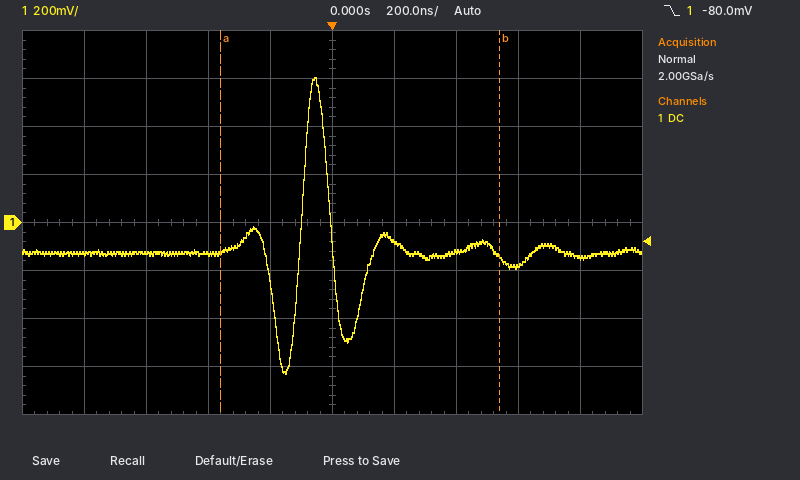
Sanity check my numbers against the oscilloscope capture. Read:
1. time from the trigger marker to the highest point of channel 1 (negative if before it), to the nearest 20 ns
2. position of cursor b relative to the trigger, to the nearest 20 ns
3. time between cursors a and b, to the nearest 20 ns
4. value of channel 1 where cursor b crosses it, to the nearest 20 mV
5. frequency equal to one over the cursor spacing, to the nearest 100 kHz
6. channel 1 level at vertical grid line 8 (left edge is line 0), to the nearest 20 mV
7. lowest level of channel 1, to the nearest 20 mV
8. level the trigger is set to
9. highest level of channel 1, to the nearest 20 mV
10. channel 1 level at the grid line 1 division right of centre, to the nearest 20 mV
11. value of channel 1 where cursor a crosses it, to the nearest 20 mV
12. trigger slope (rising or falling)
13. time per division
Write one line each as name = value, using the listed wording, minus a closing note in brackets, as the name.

time from the trigger marker to the highest point of channel 1 (negative if before it), to the nearest 20 ns = -60 ns
position of cursor b relative to the trigger, to the nearest 20 ns = +540 ns
time between cursors a and b, to the nearest 20 ns = 900 ns
value of channel 1 where cursor b crosses it, to the nearest 20 mV = -140 mV
frequency equal to one over the cursor spacing, to the nearest 100 kHz = 1.1 MHz
channel 1 level at vertical grid line 8 (left edge is line 0), to the nearest 20 mV = -180 mV
lowest level of channel 1, to the nearest 20 mV = -620 mV
level the trigger is set to = -80.0 mV
highest level of channel 1, to the nearest 20 mV = 600 mV
channel 1 level at the grid line 1 division right of centre, to the nearest 20 mV = -80 mV
value of channel 1 where cursor a crosses it, to the nearest 20 mV = -120 mV
trigger slope = falling
time per division = 200 ns
